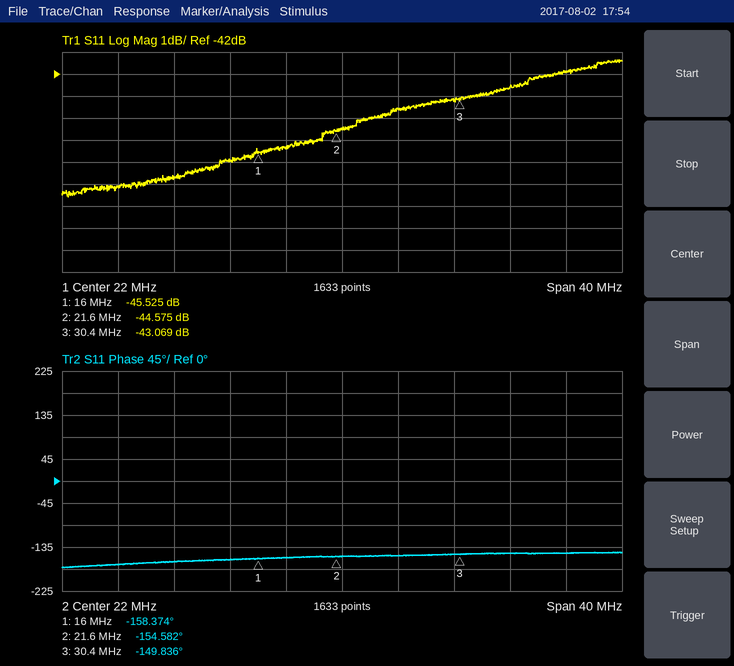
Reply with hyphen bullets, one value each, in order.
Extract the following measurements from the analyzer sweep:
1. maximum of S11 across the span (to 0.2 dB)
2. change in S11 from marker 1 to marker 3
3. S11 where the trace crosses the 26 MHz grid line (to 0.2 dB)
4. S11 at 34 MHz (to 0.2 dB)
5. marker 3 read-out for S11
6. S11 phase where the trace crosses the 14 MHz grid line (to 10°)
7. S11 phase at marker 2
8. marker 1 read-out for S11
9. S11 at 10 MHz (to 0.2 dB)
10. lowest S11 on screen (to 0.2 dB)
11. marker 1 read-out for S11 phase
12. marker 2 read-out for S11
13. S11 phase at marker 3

- -41.4 dB
- 2.456 dB
- -43.6 dB
- -42.6 dB
- -43.069 dB
- -160°
- -154.582°
- -45.525 dB
- -46.8 dB
- -47.6 dB
- -158.374°
- -44.575 dB
- -149.836°
